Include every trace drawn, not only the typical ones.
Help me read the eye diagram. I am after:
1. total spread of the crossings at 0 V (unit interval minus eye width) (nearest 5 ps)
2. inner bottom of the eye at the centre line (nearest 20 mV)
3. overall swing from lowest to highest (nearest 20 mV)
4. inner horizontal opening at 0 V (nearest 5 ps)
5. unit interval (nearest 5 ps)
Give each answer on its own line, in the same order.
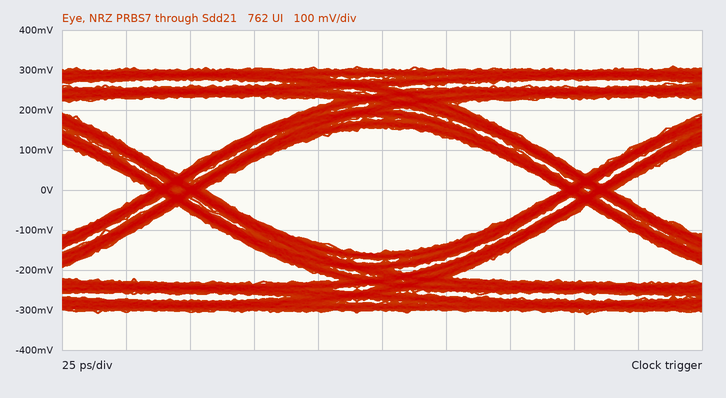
20 ps
-160 mV
620 mV
140 ps
160 ps
